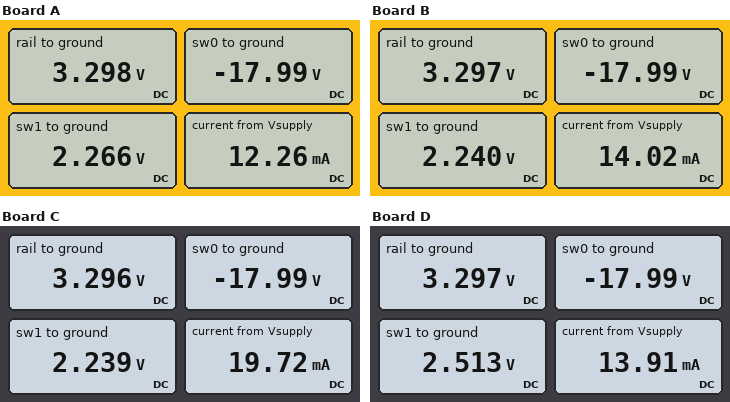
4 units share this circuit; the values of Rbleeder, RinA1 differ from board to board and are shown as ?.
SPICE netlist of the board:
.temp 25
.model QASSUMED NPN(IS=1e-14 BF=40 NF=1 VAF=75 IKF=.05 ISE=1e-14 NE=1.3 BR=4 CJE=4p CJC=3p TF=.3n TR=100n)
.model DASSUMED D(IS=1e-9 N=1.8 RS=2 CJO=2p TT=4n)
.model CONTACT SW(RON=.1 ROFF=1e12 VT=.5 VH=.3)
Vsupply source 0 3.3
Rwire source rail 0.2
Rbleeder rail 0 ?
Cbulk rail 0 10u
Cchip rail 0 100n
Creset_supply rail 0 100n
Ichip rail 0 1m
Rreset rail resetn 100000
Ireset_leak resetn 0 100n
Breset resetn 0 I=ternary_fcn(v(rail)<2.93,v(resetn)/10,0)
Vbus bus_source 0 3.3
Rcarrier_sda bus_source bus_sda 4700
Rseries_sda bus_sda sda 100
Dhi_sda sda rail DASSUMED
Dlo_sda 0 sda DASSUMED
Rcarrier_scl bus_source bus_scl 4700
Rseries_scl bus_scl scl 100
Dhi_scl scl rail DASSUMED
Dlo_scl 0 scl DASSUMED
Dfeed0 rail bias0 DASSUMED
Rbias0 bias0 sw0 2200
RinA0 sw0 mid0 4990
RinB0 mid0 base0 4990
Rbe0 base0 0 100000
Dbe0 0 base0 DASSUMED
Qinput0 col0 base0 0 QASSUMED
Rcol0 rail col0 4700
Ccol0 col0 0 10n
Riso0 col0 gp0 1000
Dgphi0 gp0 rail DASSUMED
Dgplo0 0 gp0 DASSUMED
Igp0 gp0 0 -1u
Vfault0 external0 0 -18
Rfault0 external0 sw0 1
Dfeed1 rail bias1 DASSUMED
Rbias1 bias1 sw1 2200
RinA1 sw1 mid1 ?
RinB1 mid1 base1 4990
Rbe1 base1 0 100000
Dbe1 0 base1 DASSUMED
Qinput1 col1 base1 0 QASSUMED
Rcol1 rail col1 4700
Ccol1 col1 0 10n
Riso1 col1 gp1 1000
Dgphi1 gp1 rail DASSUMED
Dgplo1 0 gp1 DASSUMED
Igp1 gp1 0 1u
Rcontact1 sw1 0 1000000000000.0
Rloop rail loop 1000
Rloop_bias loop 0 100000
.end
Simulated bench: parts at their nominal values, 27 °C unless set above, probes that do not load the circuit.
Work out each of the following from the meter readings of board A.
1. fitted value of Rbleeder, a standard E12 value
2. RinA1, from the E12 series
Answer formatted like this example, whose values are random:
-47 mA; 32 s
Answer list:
3.3 kΩ; 2.7 kΩ
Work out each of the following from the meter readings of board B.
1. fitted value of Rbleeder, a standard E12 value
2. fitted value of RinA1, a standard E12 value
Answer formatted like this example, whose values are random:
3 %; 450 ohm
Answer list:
1.2 kΩ; 2.2 kΩ
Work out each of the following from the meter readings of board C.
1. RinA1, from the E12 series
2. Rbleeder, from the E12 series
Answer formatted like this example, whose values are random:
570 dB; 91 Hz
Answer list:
2.2 kΩ; 390 Ω
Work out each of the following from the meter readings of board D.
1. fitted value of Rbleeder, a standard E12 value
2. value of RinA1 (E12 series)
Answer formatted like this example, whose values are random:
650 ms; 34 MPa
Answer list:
1.2 kΩ; 12 kΩ
